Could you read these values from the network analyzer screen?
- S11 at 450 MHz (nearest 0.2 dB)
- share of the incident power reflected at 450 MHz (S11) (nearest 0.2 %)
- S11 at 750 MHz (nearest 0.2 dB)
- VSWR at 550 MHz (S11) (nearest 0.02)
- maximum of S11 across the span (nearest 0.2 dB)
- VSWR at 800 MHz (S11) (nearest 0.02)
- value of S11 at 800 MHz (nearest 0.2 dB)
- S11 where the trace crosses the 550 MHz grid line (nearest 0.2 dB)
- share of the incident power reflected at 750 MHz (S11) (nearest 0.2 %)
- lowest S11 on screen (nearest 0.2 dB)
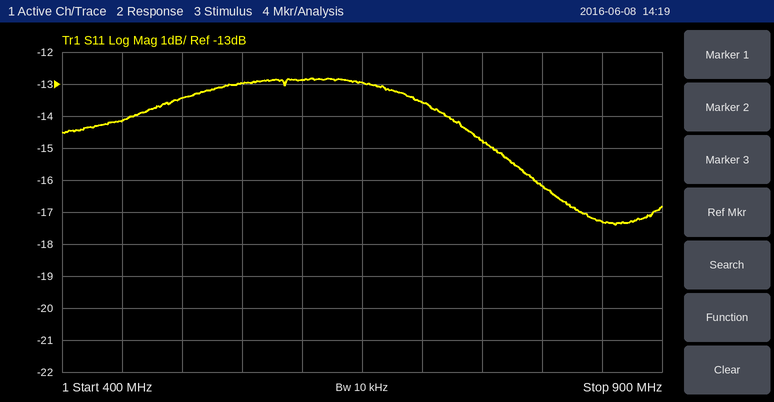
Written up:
-14.2 dB
3.8 %
-14.8 dB
1.58
-12.8 dB
1.36
-16.2 dB
-13.0 dB
3.4 %
-17.4 dB
